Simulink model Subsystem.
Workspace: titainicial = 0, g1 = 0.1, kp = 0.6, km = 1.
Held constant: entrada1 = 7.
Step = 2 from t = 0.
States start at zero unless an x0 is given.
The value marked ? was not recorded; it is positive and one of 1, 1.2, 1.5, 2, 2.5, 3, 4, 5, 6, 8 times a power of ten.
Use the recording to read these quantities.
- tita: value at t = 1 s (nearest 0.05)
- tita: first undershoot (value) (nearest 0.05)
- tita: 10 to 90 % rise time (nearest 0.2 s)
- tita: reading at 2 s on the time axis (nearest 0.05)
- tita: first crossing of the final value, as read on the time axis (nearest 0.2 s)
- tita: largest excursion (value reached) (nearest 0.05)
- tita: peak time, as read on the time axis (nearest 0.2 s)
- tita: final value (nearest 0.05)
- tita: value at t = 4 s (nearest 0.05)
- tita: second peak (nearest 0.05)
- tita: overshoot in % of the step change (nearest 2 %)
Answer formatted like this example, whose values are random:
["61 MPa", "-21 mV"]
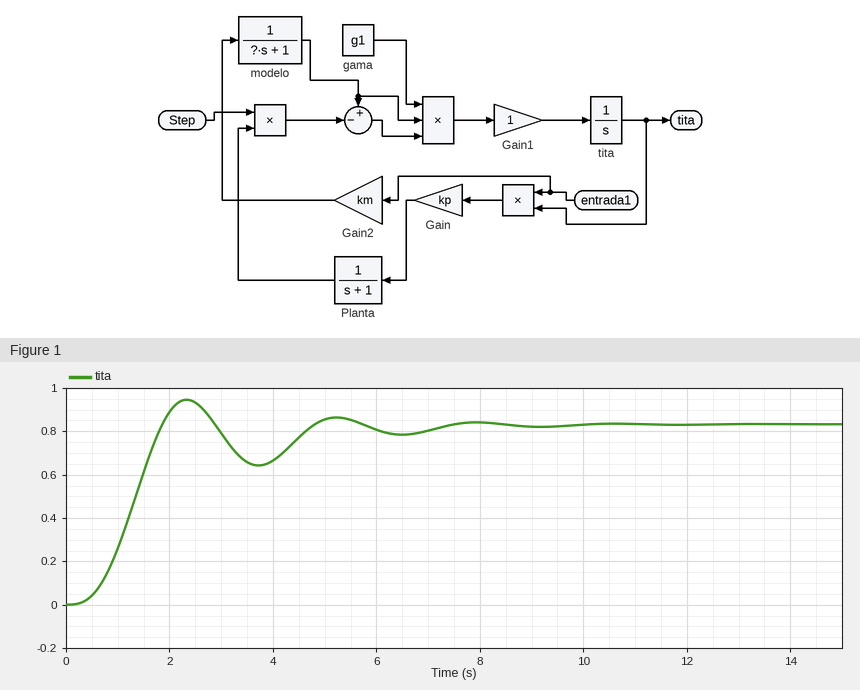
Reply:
["0.25", "0.65", "1.0 s", "0.90", "1.8 s", "0.95", "2.4 s", "0.85", "0.65", "0.85", "14 %"]
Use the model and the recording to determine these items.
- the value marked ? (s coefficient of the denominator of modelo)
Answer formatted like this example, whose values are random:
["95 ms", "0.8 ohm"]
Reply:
["2"]
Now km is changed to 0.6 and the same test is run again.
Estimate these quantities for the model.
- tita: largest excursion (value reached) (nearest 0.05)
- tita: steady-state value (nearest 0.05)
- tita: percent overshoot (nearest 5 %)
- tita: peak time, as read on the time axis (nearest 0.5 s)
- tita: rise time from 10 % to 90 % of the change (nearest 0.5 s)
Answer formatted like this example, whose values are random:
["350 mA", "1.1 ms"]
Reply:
["0.55", "0.50", "10 %", "3.0 s", "1.5 s"]
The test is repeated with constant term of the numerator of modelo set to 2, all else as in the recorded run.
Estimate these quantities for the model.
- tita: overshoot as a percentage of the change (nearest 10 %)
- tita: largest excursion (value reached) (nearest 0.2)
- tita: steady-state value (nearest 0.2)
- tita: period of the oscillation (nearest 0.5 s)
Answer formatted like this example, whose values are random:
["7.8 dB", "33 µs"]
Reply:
["20 %", "2.0", "1.6", "2.0 s"]
